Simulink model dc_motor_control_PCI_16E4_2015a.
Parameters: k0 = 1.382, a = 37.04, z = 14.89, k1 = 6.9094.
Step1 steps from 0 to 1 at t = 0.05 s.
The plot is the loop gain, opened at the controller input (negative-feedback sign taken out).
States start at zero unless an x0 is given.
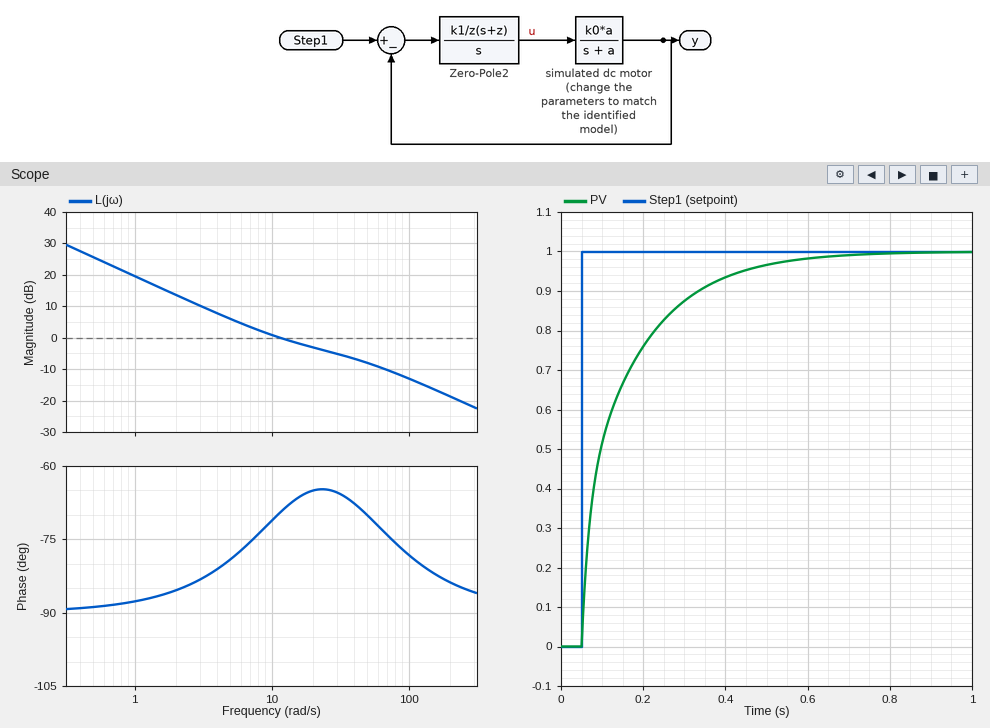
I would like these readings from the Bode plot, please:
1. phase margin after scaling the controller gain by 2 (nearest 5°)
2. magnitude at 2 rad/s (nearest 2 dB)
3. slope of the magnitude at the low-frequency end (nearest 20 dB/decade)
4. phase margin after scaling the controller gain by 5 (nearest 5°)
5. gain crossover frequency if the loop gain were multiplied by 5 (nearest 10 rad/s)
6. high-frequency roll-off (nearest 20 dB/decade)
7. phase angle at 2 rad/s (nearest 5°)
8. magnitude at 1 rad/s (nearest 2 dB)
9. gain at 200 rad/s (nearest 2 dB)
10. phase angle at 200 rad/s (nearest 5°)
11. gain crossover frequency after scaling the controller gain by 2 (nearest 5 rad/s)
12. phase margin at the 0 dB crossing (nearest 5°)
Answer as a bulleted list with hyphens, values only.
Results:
- 115°
- 14 dB
- -20 dB/decade
- 100°
- 110 rad/s
- -20 dB/decade
- -85°
- 20 dB
- -18 dB
- -85°
- 35 rad/s
- 110°
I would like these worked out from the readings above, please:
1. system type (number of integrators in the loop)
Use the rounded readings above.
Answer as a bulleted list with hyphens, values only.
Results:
- 1
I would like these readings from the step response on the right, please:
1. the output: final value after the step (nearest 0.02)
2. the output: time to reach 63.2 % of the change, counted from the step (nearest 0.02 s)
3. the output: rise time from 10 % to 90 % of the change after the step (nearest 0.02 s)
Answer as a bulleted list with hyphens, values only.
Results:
- 1.00
- 0.08 s
- 0.28 s
